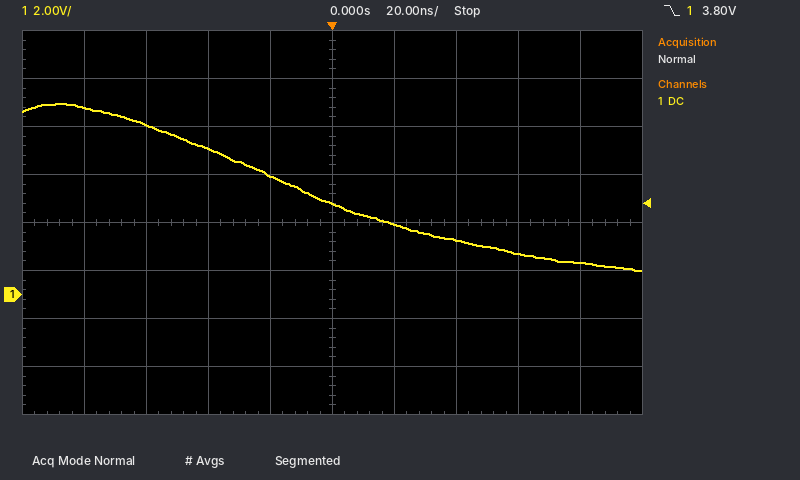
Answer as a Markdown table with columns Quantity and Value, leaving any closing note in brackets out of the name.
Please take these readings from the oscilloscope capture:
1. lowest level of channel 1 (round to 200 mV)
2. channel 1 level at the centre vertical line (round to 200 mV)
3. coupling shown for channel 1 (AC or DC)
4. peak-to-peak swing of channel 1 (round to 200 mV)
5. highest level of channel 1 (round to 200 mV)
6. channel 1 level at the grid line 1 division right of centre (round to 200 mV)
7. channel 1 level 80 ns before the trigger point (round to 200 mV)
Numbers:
| Quantity | Value |
|---|---|
| lowest level of channel 1 | 1.0 V |
| channel 1 level at the centre vertical line | 3.8 V |
| coupling shown for channel 1 | DC |
| peak-to-peak swing of channel 1 | 7.0 V |
| highest level of channel 1 | 8.0 V |
| channel 1 level at the grid line 1 division right of centre | 3.0 V |
| channel 1 level 80 ns before the trigger point | 7.8 V |
